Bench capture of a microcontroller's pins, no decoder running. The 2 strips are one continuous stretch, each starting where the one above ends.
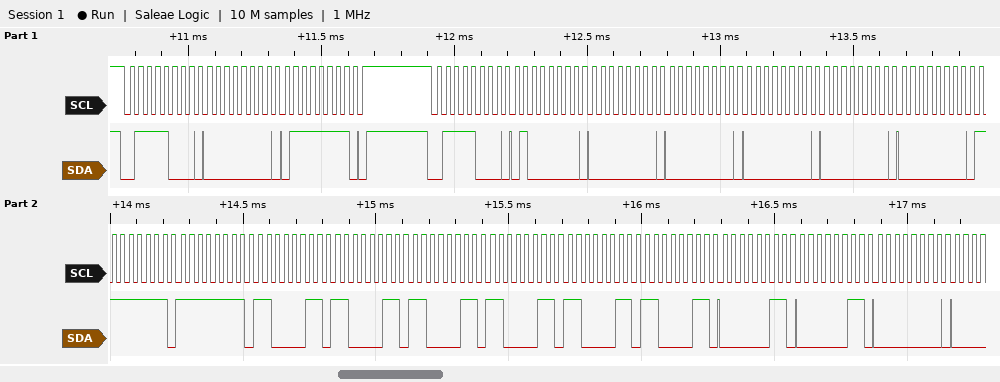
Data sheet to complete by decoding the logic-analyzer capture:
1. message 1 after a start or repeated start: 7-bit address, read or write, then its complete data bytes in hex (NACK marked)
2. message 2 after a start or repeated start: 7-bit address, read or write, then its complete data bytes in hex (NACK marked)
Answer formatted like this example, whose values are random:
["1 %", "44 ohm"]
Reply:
["0x3C write: 00 7F", "0x3C write: 40 00 00 00 00 00 FF FF C3 C3 C3 C3 C3 C3 03 03 00"]
